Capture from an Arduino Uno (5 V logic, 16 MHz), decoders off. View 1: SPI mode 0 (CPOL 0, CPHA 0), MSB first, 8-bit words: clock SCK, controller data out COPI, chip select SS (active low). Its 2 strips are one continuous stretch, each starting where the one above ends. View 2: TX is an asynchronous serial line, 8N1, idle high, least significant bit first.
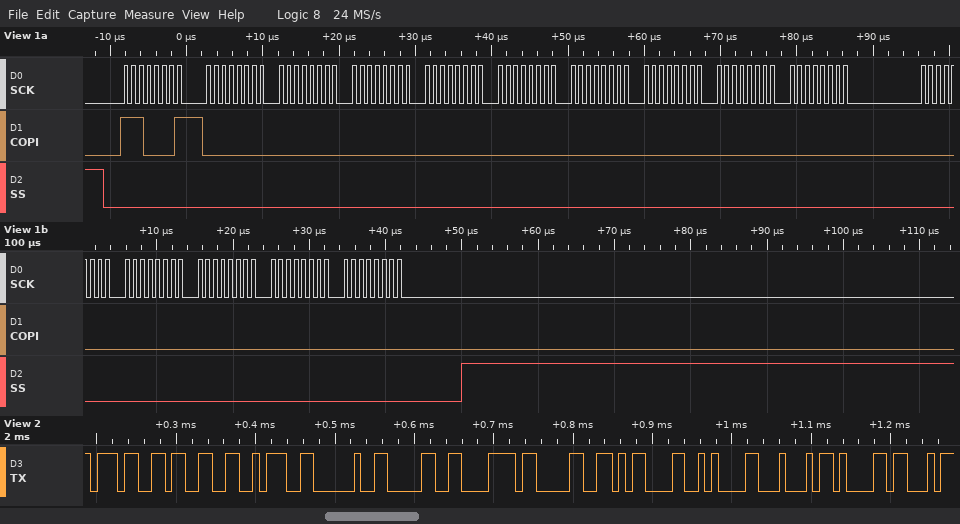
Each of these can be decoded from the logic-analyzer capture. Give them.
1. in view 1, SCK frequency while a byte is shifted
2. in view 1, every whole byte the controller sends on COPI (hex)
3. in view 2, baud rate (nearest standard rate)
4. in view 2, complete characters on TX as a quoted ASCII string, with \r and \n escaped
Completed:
1 MHz
E1 00 00 00 00 00 00 00 00 00 00 00 00 00 00
115200 baud
"73: 0x0\r\nDa"
